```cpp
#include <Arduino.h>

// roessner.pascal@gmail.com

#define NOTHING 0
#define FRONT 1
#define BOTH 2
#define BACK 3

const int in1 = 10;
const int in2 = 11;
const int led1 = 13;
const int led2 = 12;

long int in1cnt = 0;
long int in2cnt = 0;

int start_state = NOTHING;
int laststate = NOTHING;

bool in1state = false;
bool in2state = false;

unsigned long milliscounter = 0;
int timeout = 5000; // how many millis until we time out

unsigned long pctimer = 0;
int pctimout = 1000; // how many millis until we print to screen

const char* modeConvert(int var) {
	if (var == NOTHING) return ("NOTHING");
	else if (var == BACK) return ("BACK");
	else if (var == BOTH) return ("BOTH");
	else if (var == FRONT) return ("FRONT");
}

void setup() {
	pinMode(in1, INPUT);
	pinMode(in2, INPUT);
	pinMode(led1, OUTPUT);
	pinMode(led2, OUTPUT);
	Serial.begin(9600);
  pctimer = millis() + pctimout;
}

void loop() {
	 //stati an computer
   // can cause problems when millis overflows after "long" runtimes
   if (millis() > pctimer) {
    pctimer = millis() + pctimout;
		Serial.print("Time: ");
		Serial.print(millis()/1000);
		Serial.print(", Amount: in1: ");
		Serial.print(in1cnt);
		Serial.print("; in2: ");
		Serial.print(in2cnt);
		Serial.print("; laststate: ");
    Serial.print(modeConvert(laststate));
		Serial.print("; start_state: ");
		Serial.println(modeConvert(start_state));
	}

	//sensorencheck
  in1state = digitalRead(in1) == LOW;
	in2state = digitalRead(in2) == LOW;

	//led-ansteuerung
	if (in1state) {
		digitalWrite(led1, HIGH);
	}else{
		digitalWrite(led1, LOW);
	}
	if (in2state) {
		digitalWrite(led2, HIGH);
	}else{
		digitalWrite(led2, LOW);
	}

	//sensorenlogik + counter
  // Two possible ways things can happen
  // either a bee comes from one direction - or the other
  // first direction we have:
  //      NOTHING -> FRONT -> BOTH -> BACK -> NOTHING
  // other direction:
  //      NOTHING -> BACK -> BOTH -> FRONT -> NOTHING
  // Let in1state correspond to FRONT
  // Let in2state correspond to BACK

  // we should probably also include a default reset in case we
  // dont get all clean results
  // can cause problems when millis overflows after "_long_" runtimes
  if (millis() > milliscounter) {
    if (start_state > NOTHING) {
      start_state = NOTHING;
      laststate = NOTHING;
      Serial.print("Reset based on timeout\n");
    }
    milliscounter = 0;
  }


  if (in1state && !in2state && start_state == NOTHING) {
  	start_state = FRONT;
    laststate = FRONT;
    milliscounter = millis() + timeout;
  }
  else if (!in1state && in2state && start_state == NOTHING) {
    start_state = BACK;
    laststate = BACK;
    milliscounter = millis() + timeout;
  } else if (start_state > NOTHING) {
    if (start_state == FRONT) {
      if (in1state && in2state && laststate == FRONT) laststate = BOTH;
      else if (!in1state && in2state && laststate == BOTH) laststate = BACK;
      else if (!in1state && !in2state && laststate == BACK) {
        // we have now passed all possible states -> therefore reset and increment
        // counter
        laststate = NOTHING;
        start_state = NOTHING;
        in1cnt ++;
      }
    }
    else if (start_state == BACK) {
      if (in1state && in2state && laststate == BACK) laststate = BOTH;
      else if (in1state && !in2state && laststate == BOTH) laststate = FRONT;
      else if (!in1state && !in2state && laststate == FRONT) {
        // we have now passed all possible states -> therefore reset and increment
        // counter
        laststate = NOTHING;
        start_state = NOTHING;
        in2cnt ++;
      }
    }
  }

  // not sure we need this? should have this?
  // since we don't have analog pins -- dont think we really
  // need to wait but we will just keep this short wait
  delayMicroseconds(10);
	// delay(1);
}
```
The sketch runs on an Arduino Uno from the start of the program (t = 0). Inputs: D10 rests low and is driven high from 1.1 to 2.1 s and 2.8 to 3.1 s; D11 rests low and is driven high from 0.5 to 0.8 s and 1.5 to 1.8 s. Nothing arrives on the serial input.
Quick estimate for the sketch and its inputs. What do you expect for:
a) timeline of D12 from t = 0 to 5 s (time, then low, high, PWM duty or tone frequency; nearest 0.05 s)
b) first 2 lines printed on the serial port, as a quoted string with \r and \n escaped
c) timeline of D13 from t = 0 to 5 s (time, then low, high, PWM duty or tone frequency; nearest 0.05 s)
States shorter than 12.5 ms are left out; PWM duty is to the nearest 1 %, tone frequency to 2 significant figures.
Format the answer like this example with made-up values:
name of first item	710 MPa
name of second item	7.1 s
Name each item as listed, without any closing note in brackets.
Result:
timeline of D12 from t = 0 to 5 s	0 s high; 0.5 s low; 0.8 s high; 1.5 s low; 1.8 s high
first 2 lines printed on the serial port, as a quoted string with \r and \n escaped	"Time: 1, Amount: in1: 0; in2: 0; laststate: BOTH; start_state: FRONT\r\nTime: 2, Amount: in1: 1; in2: 0; laststate: BACK; start_state: BACK\r\n"
timeline of D13 from t = 0 to 5 s	0 s high; 1.1 s low; 2.1 s high; 2.8 s low; 3.1 s high
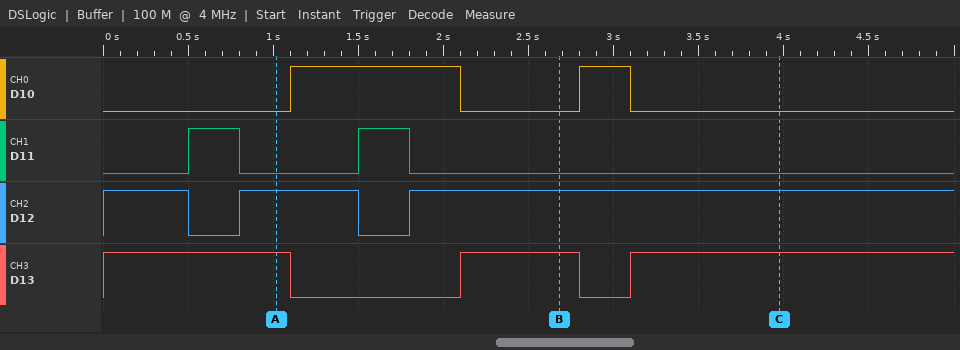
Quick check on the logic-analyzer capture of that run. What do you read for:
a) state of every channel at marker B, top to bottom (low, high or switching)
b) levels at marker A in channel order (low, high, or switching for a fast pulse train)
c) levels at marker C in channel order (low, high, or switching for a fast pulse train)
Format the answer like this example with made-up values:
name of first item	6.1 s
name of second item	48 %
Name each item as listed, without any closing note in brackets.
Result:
state of every channel at marker B, top to bottom	D10 low, D11 low, D12 high, D13 high
levels at marker A in channel order	D10 low, D11 low, D12 high, D13 high
levels at marker C in channel order	D10 low, D11 low, D12 high, D13 high
